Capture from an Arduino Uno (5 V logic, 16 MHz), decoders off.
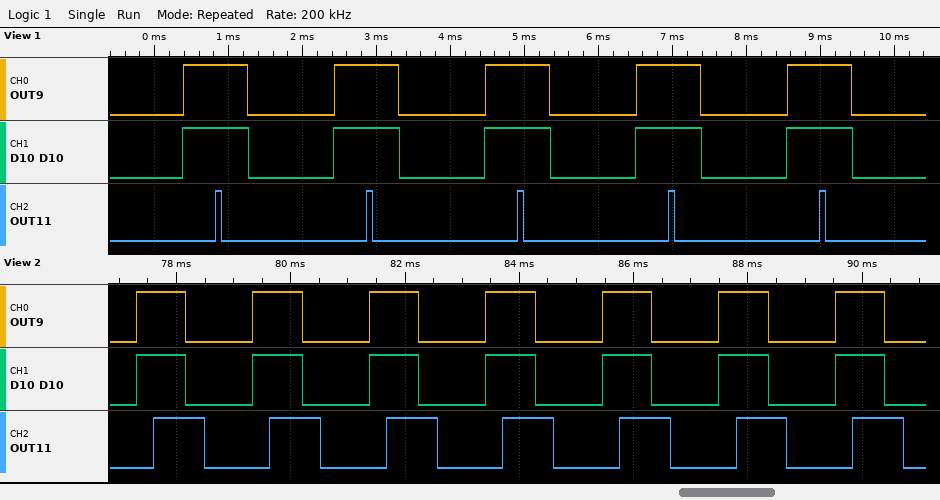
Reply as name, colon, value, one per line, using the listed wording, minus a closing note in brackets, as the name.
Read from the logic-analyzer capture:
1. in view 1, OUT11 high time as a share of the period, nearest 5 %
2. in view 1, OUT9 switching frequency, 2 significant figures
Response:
in view 1, OUT11 high time as a share of the period, nearest 5 %: 5 %
in view 1, OUT9 switching frequency, 2 significant figures: 490 Hz
